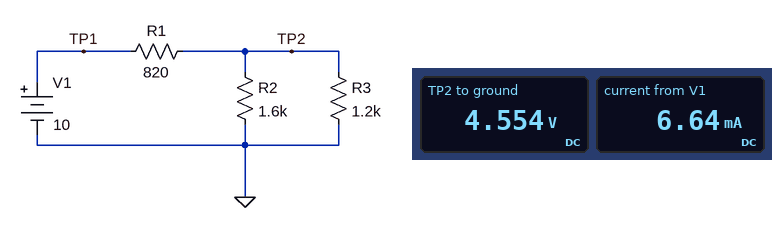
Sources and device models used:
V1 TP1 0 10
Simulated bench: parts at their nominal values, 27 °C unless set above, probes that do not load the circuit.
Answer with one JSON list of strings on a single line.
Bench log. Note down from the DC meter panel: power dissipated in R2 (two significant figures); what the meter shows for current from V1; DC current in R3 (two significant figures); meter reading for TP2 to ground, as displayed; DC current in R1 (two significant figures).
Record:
["13 mW", "6.64 mA", "3.8 mA", "4.554 V", "6.6 mA"]
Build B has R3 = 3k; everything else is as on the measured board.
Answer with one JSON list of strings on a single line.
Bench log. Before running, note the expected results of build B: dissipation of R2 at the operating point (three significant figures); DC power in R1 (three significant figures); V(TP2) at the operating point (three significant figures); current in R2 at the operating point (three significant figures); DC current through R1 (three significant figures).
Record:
["19.6 mW", "23.6 mW", "5.60 V", "3.50 mA", "5.37 mA"]
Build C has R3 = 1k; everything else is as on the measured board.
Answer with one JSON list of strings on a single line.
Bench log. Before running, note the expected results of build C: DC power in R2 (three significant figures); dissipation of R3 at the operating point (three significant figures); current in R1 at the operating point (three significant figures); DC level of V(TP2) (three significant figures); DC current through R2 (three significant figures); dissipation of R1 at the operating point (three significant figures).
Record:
["11.5 mW", "18.4 mW", "6.97 mA", "4.29 V", "2.68 mA", "39.8 mW"]
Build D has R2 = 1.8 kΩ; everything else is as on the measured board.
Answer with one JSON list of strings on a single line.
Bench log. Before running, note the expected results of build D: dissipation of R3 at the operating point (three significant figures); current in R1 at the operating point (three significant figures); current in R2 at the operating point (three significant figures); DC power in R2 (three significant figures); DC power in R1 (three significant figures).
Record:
["18.2 mW", "6.49 mA", "2.60 mA", "12.1 mW", "34.6 mW"]
